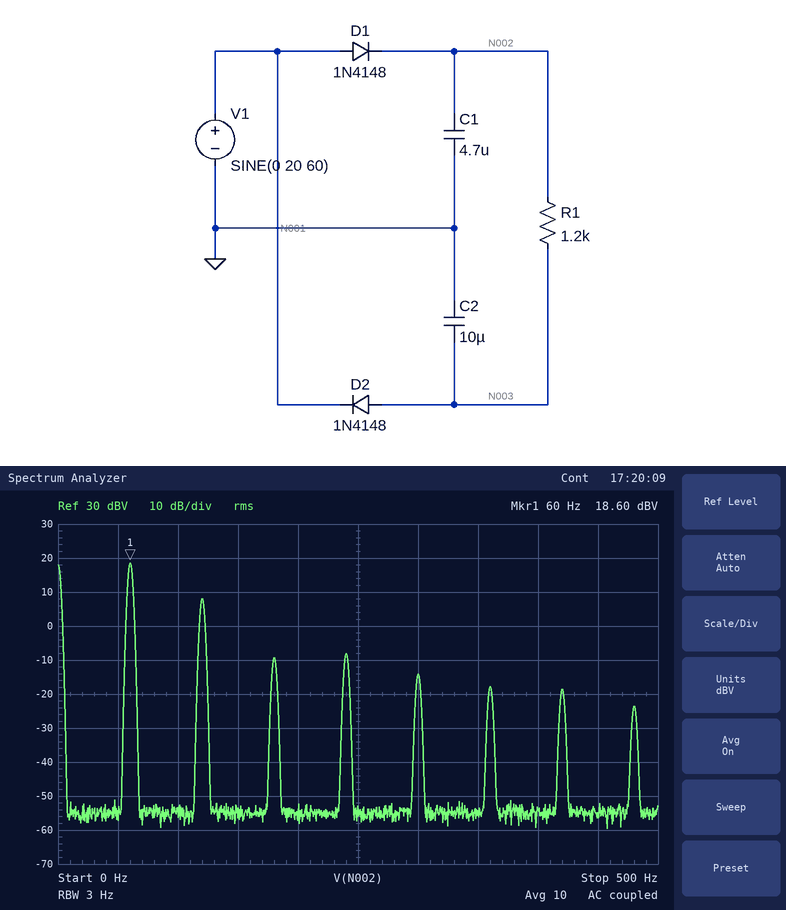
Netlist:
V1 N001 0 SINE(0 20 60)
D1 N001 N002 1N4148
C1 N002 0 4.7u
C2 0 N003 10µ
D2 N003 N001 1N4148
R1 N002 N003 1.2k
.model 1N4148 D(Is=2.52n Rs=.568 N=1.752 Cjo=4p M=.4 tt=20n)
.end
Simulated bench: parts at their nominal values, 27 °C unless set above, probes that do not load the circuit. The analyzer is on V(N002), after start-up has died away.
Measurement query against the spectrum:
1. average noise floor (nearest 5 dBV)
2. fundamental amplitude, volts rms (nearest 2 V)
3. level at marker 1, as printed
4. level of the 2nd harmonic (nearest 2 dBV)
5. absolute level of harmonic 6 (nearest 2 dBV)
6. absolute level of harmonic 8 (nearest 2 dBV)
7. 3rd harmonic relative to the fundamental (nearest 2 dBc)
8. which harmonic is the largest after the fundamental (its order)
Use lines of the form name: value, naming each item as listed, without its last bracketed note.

average noise floor: -55 dBV
fundamental amplitude, volts rms: 8 V
level at marker 1, as printed: 18.60 dBV
level of the 2nd harmonic: 8 dBV
absolute level of harmonic 6: -18 dBV
absolute level of harmonic 8: -24 dBV
3rd harmonic relative to the fundamental: -28 dBc
which harmonic is the largest after the fundamental: 2
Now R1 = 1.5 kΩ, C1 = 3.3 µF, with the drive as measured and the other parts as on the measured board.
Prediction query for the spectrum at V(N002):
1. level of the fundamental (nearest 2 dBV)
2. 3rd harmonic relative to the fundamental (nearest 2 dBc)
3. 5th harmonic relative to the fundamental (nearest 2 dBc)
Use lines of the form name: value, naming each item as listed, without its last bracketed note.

level of the fundamental: 20 dBV
3rd harmonic relative to the fundamental: -32 dBc
5th harmonic relative to the fundamental: -34 dBc
